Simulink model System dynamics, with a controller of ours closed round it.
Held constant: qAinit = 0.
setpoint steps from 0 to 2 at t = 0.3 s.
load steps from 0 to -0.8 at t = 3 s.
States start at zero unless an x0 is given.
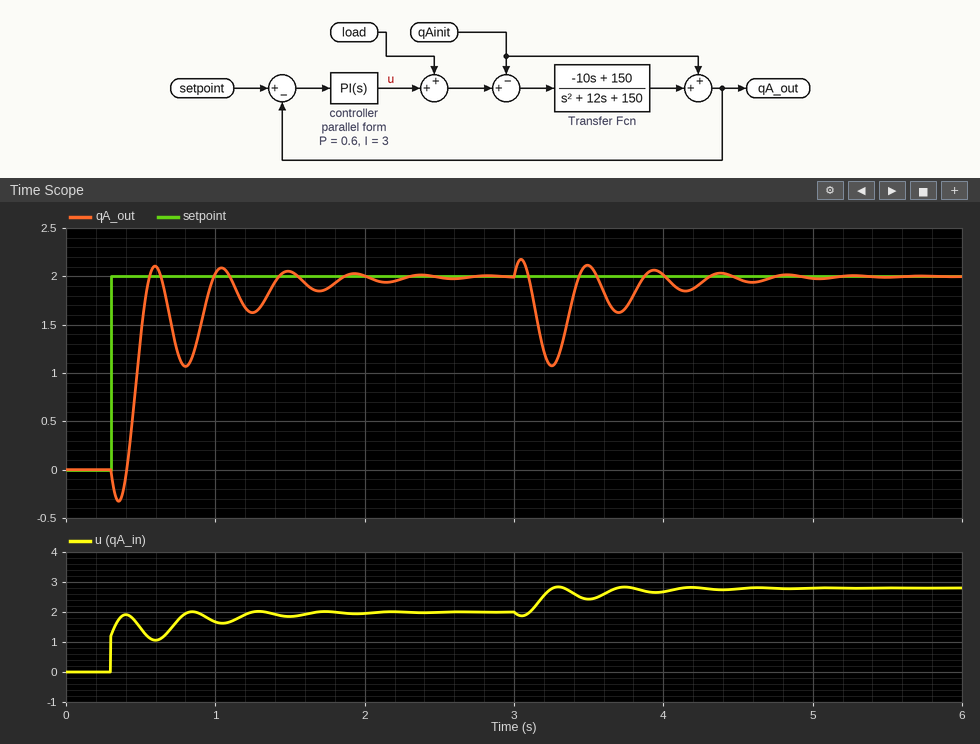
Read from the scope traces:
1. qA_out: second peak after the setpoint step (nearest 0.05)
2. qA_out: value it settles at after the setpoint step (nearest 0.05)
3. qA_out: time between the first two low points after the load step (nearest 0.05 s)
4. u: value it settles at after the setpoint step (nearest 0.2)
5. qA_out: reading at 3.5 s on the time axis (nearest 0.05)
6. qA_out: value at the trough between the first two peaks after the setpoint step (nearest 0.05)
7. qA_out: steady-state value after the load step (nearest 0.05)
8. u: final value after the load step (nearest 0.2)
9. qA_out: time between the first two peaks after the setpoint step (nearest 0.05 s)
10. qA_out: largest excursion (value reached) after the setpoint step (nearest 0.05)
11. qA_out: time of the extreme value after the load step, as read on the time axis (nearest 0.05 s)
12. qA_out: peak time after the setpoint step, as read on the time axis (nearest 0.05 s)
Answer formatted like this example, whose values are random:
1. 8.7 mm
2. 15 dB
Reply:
1. 2.10
2. 2.00
3. 0.45 s
4. 2.0
5. 2.10
6. 1.05
7. 2.00
8. 2.8
9. 0.45 s
10. 2.10
11. 3.25 s
12. 0.60 s
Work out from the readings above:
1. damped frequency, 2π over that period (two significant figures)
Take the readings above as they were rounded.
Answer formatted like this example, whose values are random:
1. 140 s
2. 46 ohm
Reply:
1. 14 rad/s
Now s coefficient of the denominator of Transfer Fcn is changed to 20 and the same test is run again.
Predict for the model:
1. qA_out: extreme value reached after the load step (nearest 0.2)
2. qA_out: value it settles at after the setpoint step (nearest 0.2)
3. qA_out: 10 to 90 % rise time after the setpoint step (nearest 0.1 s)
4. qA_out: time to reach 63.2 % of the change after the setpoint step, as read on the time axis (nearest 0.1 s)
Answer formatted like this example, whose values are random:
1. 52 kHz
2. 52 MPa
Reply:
1. 1.4
2. 2.0
3. 0.6 s
4. 0.5 s
